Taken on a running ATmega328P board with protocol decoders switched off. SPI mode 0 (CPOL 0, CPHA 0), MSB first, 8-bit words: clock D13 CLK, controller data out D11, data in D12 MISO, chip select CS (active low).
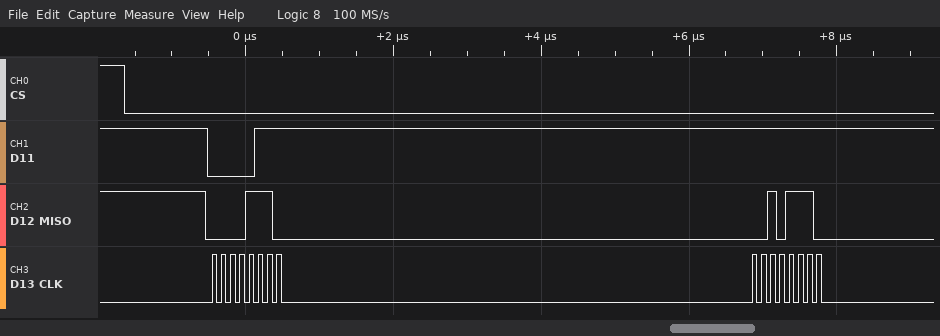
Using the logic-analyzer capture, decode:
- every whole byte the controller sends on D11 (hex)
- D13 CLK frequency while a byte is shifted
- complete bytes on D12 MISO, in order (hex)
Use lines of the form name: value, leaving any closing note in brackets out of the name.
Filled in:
every whole byte the controller sends on D11: 07 FF
D13 CLK frequency while a byte is shifted: 8 MHz
complete bytes on D12 MISO, in order: 0E 2E
